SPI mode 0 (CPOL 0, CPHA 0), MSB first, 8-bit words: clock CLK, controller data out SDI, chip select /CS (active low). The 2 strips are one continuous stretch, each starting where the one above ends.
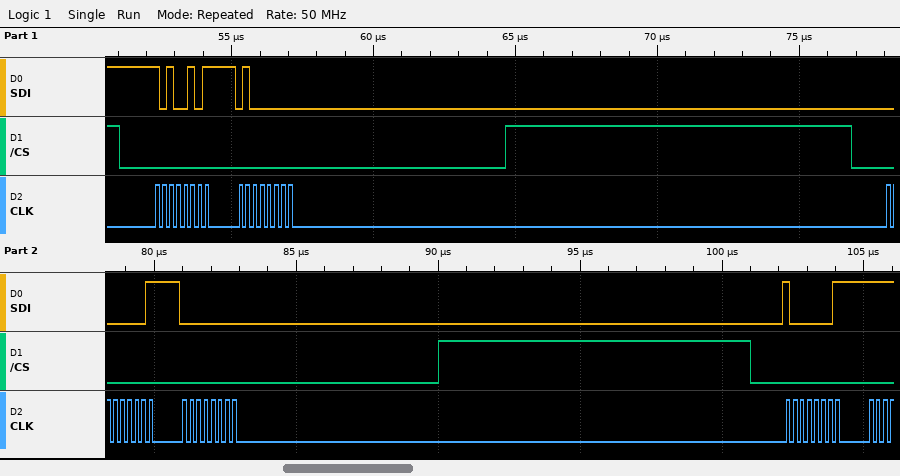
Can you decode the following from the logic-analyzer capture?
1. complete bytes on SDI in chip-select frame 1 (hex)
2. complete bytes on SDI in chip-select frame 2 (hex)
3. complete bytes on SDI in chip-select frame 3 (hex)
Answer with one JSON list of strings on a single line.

["A5 40", "01 00", "81"]
